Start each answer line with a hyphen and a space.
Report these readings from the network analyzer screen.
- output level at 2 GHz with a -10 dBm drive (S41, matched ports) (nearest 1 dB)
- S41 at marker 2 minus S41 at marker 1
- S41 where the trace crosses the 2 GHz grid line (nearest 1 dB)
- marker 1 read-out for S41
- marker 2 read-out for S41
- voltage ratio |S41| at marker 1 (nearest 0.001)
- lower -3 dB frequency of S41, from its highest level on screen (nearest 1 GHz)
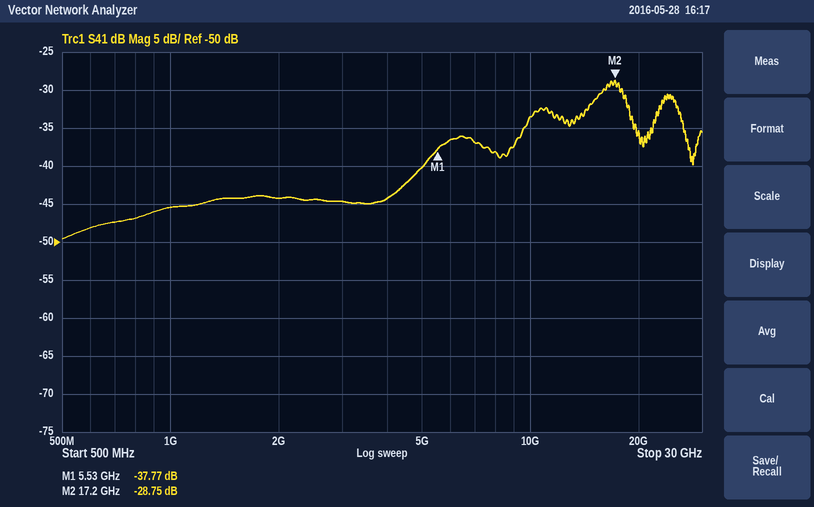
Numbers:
- -54 dBm
- 9.02 dB
- -44 dB
- -37.77 dB
- -28.75 dB
- 0.013
- 15 GHz
